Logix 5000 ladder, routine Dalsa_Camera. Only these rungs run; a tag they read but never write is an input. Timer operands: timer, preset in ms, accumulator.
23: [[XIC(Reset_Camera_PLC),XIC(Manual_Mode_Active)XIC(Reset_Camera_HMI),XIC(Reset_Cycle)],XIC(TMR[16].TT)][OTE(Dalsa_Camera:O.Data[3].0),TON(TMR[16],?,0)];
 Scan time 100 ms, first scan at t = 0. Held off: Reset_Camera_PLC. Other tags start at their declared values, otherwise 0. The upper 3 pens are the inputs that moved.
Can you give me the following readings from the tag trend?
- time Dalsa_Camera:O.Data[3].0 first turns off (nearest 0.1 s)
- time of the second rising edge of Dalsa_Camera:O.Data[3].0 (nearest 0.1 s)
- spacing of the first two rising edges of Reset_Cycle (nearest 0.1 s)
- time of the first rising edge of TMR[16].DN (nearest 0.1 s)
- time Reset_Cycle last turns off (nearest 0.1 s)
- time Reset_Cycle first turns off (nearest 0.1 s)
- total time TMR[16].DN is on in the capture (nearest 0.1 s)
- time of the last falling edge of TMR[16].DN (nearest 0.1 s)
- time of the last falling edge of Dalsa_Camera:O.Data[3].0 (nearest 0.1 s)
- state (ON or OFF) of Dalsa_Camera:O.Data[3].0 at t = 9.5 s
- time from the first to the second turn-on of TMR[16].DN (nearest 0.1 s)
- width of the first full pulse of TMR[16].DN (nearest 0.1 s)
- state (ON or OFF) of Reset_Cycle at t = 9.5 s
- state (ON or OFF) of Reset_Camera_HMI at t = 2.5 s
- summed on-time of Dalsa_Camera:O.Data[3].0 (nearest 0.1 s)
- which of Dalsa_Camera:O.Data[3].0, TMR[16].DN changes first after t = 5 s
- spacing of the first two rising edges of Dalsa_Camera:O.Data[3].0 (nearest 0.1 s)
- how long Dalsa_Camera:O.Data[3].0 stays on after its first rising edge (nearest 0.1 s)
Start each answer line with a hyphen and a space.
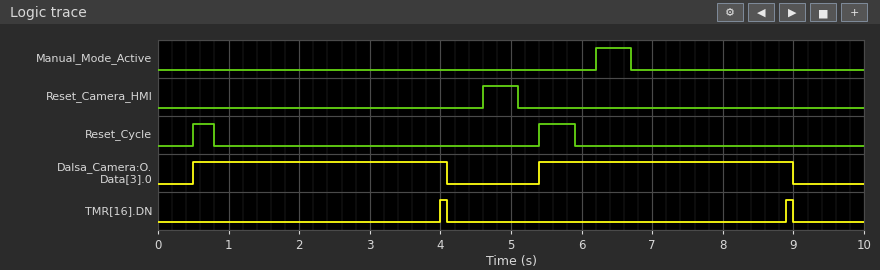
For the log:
- 4.1 s
- 5.4 s
- 4.9 s
- 4.0 s
- 5.9 s
- 0.8 s
- 0.2 s
- 9.0 s
- 9.0 s
- OFF
- 4.9 s
- 0.1 s
- OFF
- OFF
- 7.2 s
- Dalsa_Camera:O.Data[3].0
- 4.9 s
- 3.6 s
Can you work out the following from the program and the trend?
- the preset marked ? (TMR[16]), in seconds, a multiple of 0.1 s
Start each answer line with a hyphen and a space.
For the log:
- 3.5 s
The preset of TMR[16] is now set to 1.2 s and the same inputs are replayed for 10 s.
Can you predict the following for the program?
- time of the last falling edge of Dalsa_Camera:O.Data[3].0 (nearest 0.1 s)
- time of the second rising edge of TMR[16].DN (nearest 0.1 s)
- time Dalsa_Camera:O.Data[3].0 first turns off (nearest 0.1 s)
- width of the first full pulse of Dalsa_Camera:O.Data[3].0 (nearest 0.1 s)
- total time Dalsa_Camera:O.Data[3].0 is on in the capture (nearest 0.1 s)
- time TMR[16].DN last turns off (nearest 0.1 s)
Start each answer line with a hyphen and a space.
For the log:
- 6.7 s
- 6.6 s
- 1.8 s
- 1.3 s
- 2.6 s
- 6.7 s
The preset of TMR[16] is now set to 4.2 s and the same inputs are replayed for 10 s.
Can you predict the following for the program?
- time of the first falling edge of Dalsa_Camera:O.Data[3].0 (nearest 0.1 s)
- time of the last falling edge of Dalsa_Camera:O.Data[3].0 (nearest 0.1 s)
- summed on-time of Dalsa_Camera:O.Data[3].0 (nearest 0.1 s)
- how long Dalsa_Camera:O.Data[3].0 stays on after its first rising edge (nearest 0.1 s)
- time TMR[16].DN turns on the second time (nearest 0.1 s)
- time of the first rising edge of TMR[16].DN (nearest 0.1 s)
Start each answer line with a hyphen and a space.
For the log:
- 4.8 s
- 9.7 s
- 8.6 s
- 4.3 s
- 9.6 s
- 4.7 s
